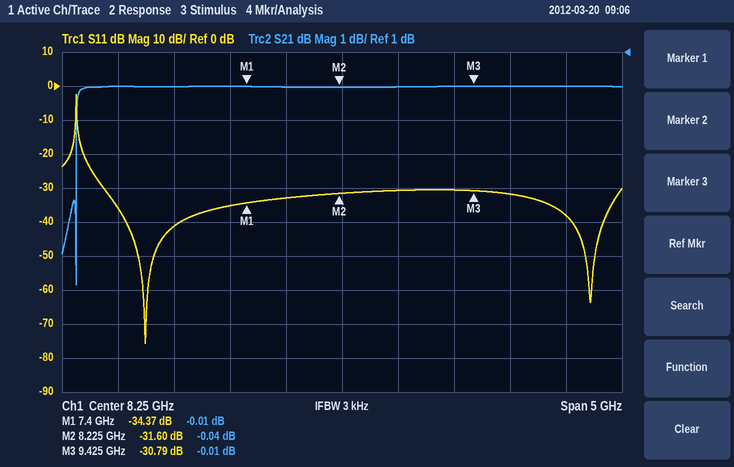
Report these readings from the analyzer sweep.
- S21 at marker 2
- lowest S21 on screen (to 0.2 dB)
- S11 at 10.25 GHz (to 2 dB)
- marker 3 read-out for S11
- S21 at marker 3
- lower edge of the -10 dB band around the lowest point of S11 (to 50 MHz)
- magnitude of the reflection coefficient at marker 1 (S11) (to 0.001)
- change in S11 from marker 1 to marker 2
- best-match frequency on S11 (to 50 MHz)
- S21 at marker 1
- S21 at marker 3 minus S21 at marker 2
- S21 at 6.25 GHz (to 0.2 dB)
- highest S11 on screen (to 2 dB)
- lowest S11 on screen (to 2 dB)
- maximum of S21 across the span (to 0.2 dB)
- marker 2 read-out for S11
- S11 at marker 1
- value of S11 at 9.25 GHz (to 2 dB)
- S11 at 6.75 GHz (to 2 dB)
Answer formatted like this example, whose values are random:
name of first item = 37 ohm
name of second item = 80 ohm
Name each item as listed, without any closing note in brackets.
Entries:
S21 at marker 2 = -0.04 dB
lowest S21 on screen = -5.8 dB
S11 at 10.25 GHz = -38 dB
marker 3 read-out for S11 = -30.79 dB
S21 at marker 3 = -0.01 dB
lower edge of the -10 dB band around the lowest point of S11 = 5.90 GHz
magnitude of the reflection coefficient at marker 1 (S11) = 0.019
change in S11 from marker 1 to marker 2 = 2.77 dB
best-match frequency on S11 = 6.50 GHz
S21 at marker 1 = -0.01 dB
S21 at marker 3 minus S21 at marker 2 = 0.03 dB
S21 at 6.25 GHz = 0.0 dB
highest S11 on screen = -2 dB
lowest S11 on screen = -76 dB
maximum of S21 across the span = 0.0 dB
marker 2 read-out for S11 = -31.60 dB
S11 at marker 1 = -34.37 dB
value of S11 at 9.25 GHz = -30 dB
S11 at 6.75 GHz = -42 dB
